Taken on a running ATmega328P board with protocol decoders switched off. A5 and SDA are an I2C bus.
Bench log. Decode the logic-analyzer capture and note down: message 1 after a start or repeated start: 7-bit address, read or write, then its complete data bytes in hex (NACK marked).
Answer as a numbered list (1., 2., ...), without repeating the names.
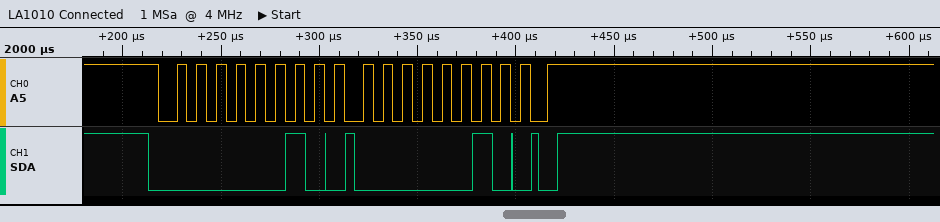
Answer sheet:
1. 0x01 write: 02
